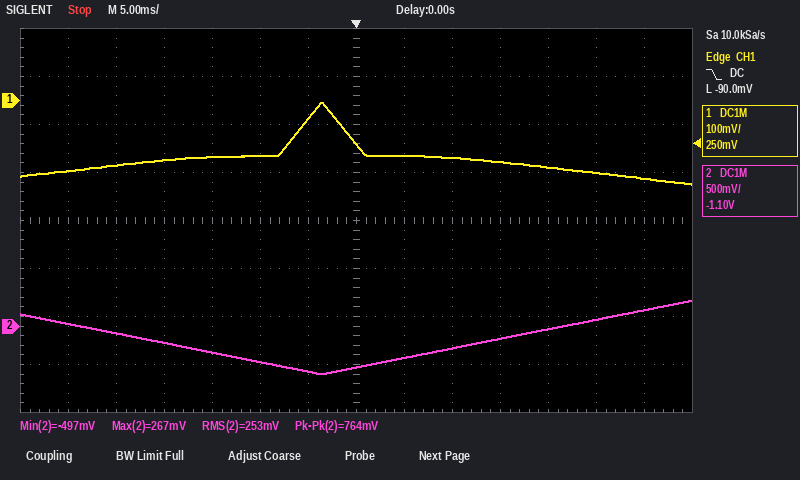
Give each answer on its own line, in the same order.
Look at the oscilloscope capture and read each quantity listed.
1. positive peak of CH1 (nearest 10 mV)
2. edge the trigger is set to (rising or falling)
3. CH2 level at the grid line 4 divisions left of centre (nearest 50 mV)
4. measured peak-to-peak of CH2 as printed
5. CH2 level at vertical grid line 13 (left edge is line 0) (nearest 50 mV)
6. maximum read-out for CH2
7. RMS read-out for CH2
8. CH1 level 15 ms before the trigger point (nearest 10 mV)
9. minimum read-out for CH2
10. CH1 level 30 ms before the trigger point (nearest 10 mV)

0 mV
falling
-150 mV
764 mV
150 mV
267 mV
253 mV
-120 mV
-497 mV
-150 mV
